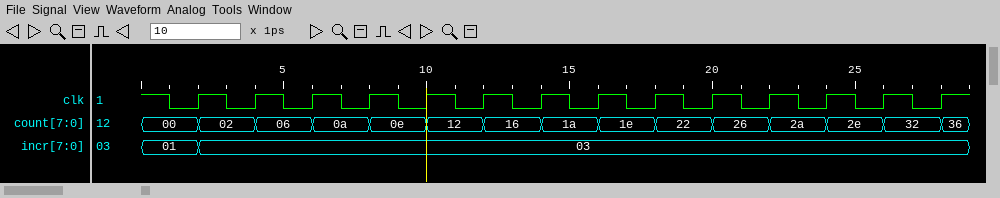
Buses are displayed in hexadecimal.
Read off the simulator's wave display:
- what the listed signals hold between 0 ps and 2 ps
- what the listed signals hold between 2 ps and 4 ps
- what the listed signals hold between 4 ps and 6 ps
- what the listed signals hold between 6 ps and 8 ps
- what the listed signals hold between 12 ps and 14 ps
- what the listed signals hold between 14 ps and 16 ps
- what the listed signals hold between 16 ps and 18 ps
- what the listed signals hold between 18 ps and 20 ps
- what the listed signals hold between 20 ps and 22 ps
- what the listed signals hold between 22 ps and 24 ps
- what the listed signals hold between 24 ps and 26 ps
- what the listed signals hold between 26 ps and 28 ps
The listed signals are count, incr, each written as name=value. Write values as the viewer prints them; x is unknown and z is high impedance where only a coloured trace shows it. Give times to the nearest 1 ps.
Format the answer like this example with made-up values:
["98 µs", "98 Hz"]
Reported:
["count=00, incr=01", "count=02, incr=03", "count=06, incr=03", "count=0a, incr=03", "count=16, incr=03", "count=1a, incr=03", "count=1e, incr=03", "count=22, incr=03", "count=26, incr=03", "count=2a, incr=03", "count=2e, incr=03", "count=32, incr=03"]
